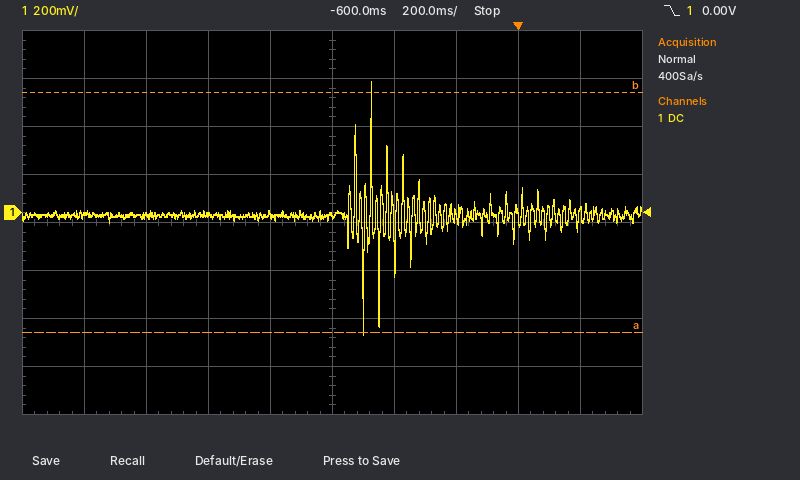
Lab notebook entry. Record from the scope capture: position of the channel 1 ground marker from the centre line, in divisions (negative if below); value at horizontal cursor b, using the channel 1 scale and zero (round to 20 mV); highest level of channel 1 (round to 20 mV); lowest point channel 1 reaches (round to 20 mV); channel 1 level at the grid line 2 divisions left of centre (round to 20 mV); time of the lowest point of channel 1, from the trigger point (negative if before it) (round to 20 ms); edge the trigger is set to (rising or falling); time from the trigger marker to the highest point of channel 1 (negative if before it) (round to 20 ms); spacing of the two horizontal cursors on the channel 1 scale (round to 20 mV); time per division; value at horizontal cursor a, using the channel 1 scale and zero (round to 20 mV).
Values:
+0.2 div
500 mV
540 mV
-500 mV
0 mV
-500 ms
falling
-480 ms
1.00 V
200 ms
-500 mV
